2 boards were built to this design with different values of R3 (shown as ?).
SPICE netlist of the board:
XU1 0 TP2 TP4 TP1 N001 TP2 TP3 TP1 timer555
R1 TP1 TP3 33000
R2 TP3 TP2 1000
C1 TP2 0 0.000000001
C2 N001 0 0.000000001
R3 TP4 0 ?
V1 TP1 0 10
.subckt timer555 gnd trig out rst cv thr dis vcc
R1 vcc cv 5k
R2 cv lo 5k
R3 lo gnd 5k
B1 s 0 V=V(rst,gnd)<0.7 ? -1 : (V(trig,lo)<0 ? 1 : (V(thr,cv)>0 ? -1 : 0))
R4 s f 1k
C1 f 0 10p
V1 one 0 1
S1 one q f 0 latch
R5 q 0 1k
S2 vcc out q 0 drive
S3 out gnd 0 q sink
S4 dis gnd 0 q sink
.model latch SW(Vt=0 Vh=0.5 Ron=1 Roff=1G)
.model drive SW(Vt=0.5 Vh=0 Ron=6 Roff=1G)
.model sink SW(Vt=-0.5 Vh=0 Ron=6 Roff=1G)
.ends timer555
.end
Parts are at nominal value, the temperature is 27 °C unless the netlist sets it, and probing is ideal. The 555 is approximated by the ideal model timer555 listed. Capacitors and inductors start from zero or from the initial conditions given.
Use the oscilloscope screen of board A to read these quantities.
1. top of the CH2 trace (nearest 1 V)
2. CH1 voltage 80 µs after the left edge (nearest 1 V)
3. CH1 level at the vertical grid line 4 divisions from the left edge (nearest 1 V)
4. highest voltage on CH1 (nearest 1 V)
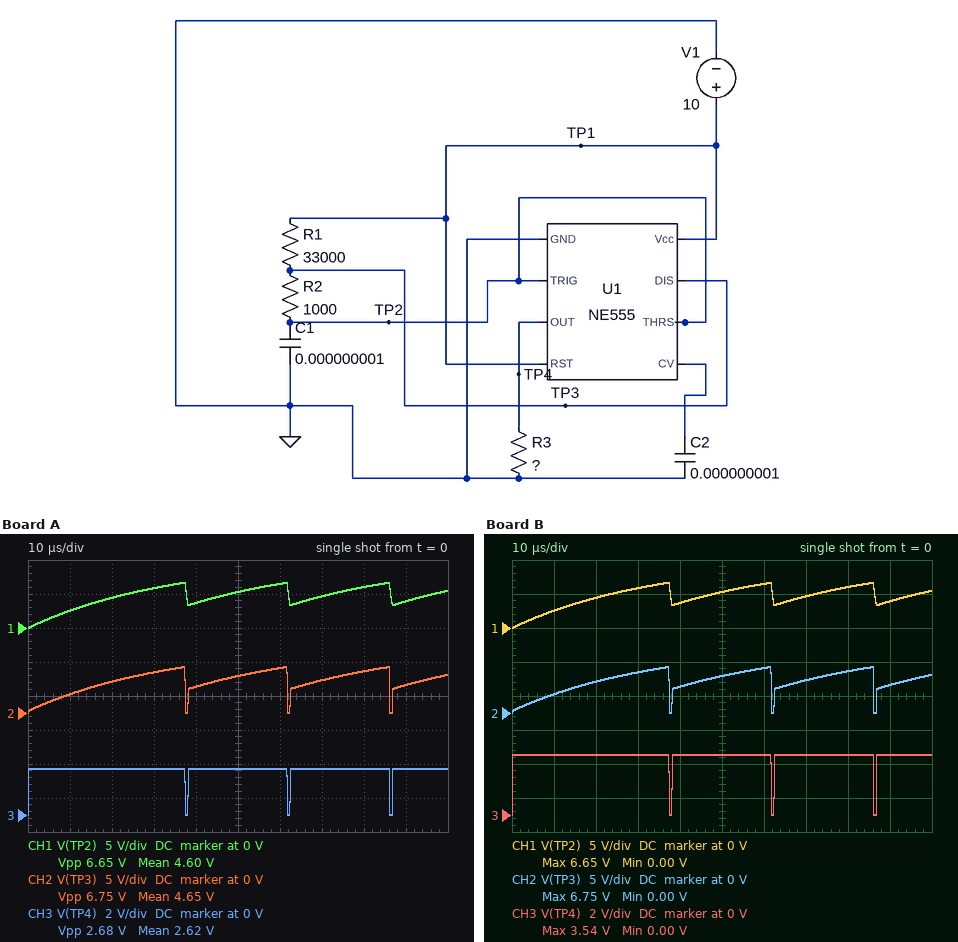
7 V
6 V
4 V
7 V
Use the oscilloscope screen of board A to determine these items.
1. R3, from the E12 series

2.2 Ω
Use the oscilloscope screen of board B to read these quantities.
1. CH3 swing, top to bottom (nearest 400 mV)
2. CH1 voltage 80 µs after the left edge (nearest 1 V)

3.6 V
6 V
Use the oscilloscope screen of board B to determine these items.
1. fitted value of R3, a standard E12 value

3.3 Ω
